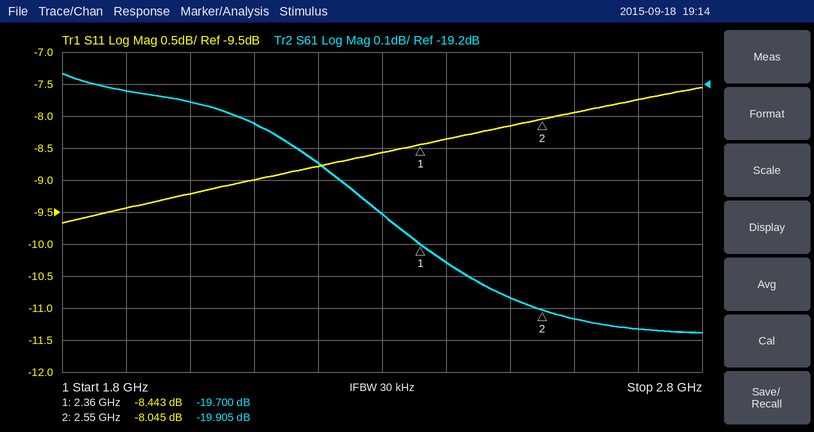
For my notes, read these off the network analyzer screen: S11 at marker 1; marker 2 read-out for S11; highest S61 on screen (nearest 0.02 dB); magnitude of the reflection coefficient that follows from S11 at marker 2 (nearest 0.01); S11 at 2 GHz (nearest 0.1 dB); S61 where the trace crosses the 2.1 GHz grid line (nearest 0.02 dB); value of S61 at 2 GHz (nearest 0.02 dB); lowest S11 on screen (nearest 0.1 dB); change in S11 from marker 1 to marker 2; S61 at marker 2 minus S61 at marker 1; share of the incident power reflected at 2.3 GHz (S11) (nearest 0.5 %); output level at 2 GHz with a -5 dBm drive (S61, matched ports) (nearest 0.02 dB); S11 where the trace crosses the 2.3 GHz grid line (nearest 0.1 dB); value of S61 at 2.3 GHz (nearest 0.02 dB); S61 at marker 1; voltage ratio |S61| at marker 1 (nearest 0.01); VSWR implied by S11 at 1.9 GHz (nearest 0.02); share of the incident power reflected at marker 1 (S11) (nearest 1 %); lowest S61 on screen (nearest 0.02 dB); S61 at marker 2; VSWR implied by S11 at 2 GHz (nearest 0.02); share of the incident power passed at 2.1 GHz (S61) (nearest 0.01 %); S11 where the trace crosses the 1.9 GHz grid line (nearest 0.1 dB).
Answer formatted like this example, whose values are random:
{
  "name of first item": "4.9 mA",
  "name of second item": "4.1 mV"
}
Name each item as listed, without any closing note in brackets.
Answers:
{
  "S11 at marker 1": "-8.443 dB",
  "marker 2 read-out for S11": "-8.045 dB",
  "highest S61 on screen": "-19.16 dB",
  "magnitude of the reflection coefficient that follows from S11 at marker 2": "0.40",
  "S11 at 2 GHz": "-9.2 dB",
  "S61 where the trace crosses the 2.1 GHz grid line": "-19.32 dB",
  "value of S61 at 2 GHz": "-19.26 dB",
  "lowest S11 on screen": "-9.7 dB",
  "change in S11 from marker 1 to marker 2": "0.398 dB",
  "S61 at marker 2 minus S61 at marker 1": "-0.205 dB",
  "share of the incident power reflected at 2.3 GHz (S11)": "14.0 %",
  "output level at 2 GHz with a -5 dBm drive (S61, matched ports)": "-24.26 dBm",
  "S11 where the trace crosses the 2.3 GHz grid line": "-8.6 dB",
  "value of S61 at 2.3 GHz": "-19.60 dB",
  "S61 at marker 1": "-19.700 dB",
  "voltage ratio |S61| at marker 1": "0.10",
  "VSWR implied by S11 at 1.9 GHz": "2.02",
  "share of the incident power reflected at marker 1 (S11)": "14 %",
  "lowest S61 on screen": "-19.98 dB",
  "S61 at marker 2": "-19.905 dB",
  "VSWR implied by S11 at 2 GHz": "2.06",
  "share of the incident power passed at 2.1 GHz (S61)": "1.17 %",
  "S11 where the trace crosses the 1.9 GHz grid line": "-9.4 dB"
}
